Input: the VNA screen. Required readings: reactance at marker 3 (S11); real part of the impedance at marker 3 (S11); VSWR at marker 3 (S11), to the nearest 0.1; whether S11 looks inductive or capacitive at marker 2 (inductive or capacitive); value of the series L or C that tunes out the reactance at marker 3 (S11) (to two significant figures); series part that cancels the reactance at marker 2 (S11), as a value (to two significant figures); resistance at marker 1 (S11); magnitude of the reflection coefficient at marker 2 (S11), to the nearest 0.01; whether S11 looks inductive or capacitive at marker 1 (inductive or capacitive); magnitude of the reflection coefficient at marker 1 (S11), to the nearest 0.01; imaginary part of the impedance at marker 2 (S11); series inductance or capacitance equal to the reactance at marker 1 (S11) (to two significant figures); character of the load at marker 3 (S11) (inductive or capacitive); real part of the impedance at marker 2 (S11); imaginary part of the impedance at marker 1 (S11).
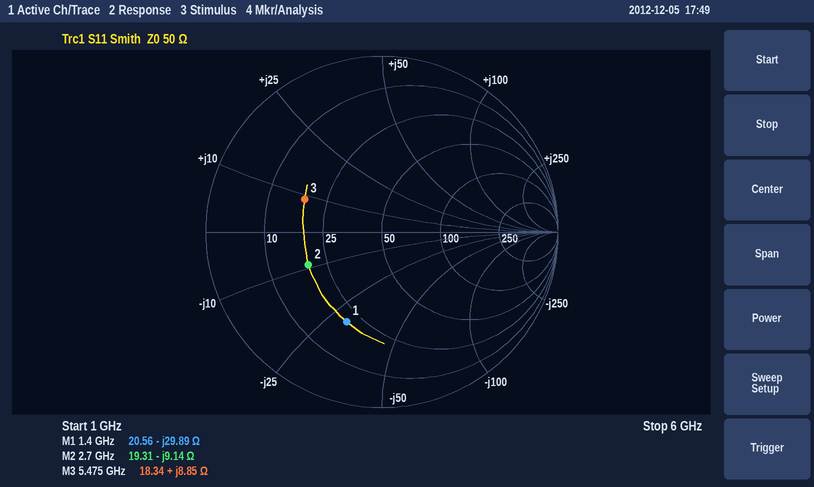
+8.85 Ω
18.34 Ω
2.8
capacitive
3.3 pF
540 pH
20.56 Ω
0.46
capacitive
0.55
-9.14 Ω
3.8 pF
inductive
19.31 Ω
-29.89 Ω
